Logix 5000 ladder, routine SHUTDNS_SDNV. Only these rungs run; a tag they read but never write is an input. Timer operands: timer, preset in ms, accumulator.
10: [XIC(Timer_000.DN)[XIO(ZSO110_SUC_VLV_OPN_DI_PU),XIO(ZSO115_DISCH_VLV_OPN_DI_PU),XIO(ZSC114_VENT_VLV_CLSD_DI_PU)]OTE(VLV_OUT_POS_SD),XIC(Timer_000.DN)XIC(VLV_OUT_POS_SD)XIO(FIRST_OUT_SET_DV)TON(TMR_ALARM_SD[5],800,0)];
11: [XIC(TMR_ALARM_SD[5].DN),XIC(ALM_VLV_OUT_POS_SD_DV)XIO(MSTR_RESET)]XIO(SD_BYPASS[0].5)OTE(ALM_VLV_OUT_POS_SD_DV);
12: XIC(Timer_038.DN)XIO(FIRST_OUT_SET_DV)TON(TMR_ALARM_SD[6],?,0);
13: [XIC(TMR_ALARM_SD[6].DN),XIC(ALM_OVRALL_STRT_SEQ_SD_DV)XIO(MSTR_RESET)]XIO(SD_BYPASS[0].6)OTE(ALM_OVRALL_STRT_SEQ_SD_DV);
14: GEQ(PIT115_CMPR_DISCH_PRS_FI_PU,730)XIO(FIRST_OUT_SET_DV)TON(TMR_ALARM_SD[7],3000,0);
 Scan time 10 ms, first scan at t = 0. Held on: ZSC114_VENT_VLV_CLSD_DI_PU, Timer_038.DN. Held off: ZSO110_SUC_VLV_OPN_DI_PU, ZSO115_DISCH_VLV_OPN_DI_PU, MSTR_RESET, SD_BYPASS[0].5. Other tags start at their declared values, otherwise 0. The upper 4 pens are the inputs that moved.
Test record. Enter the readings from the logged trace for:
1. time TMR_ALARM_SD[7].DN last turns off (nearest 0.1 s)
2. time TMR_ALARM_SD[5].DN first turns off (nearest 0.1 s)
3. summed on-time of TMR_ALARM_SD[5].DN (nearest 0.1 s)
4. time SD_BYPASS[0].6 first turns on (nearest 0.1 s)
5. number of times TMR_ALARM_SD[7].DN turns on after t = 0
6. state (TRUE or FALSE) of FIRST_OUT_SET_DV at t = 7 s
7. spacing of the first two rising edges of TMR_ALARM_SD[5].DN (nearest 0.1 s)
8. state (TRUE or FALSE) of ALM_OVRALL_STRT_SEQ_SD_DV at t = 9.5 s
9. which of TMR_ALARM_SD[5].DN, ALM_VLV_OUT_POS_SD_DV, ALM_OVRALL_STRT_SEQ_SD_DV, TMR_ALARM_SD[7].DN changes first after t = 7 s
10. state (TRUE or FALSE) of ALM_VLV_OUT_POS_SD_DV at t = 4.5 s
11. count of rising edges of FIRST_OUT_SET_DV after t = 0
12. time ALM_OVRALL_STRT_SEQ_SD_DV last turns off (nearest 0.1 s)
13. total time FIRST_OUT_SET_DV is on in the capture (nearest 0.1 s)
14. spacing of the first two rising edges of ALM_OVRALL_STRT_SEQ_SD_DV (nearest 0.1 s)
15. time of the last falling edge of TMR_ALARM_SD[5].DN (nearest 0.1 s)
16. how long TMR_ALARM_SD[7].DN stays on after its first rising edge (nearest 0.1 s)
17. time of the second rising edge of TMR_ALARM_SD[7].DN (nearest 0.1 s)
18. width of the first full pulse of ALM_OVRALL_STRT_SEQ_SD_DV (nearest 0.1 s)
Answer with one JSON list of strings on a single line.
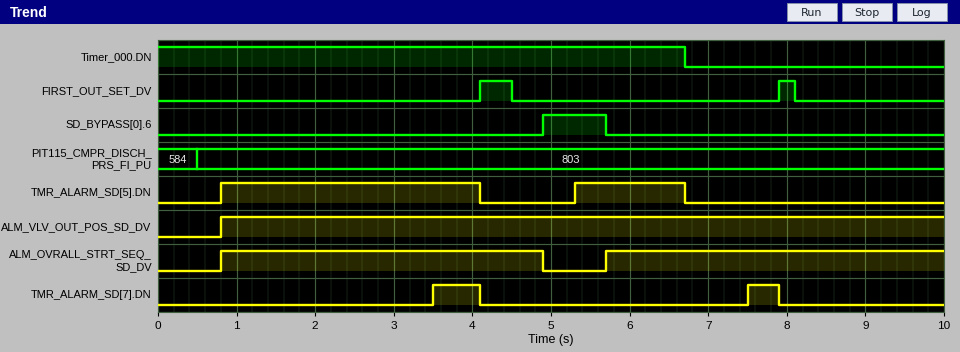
["7.9 s", "4.1 s", "4.7 s", "4.9 s", "2", "FALSE", "4.5 s", "TRUE", "TMR_ALARM_SD[7].DN", "TRUE", "2", "4.9 s", "0.6 s", "4.9 s", "6.7 s", "0.6 s", "7.5 s", "4.1 s"]
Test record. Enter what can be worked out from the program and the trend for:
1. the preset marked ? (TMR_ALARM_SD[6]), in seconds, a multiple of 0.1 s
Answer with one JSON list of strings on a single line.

["0.8 s"]
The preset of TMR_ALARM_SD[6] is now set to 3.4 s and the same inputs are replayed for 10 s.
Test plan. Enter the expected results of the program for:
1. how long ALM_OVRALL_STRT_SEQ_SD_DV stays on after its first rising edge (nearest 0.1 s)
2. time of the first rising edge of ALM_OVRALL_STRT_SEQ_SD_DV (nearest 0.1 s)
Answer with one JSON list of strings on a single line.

["1.5 s", "3.4 s"]
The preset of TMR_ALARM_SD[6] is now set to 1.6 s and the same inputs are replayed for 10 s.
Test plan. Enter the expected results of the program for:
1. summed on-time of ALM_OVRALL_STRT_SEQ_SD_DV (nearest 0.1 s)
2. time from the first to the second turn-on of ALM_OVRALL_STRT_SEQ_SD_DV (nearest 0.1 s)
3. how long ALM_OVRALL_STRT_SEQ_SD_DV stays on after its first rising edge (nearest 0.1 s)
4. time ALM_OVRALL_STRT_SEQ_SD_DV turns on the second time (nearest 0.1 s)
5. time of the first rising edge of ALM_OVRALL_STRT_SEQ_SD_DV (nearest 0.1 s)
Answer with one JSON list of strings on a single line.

["7.2 s", "4.5 s", "3.3 s", "6.1 s", "1.6 s"]
